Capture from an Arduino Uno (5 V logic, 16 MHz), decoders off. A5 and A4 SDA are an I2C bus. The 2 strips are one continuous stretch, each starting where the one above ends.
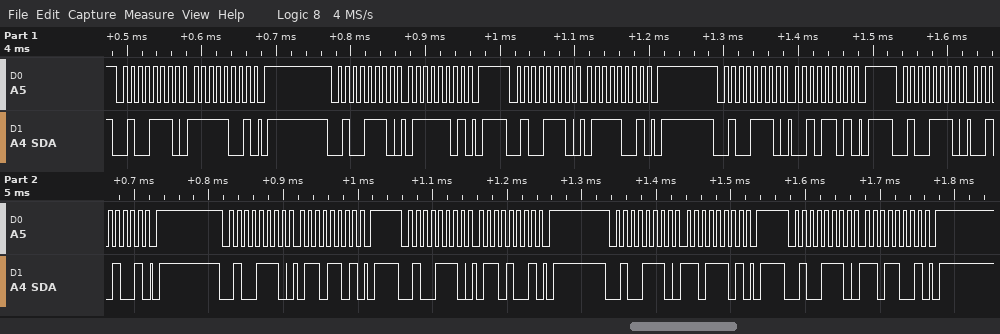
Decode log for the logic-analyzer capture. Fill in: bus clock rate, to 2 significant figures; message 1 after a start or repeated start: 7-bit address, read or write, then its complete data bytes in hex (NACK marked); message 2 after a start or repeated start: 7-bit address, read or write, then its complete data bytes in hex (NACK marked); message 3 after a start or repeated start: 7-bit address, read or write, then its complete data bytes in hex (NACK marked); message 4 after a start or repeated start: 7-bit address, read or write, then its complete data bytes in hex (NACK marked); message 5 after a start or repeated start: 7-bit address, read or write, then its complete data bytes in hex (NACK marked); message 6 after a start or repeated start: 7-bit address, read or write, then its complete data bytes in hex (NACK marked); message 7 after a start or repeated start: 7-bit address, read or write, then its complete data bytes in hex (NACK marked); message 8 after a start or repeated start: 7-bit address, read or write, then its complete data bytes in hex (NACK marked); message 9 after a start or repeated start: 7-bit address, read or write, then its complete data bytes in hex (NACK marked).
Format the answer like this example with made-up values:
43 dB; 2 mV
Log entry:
100 kHz; 0x27 write: F9; 0x27 write: 7D; 0x27 write: 79; 0x27 write: 2D; 0x27 write: 29; 0x27 write: 6D; 0x27 write: 69; 0x27 write: DD; 0x27 write: D9
